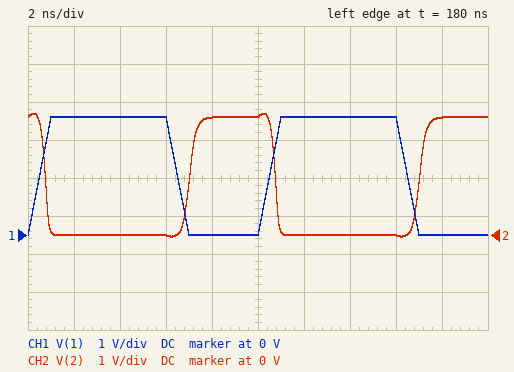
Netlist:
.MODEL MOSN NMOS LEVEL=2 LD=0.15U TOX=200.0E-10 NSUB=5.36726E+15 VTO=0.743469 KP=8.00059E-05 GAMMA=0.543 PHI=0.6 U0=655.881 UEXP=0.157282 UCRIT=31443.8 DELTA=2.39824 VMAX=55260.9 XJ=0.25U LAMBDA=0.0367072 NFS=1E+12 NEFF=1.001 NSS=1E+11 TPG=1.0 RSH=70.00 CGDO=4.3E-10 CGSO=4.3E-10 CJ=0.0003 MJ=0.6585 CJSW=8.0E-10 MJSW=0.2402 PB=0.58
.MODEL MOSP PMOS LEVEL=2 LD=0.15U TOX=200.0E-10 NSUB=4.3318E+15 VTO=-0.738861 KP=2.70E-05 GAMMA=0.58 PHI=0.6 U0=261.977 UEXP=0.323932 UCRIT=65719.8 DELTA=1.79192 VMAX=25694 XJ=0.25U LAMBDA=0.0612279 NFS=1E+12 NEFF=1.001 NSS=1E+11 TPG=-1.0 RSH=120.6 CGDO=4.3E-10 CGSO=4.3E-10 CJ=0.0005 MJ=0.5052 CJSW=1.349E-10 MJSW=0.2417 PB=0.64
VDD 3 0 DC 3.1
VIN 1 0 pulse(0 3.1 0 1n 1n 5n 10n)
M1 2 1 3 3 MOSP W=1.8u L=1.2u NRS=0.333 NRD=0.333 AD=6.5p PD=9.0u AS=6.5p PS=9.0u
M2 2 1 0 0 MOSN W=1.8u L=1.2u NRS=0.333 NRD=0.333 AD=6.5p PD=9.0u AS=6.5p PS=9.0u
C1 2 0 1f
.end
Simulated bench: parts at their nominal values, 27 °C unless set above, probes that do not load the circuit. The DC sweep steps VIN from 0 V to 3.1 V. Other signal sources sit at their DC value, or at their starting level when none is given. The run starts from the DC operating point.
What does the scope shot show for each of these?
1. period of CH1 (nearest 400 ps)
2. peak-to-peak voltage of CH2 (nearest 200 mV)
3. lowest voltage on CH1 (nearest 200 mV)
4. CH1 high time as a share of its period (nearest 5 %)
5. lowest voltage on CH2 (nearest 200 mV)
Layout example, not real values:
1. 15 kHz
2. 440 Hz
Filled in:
1. 10.0 ns
2. 3.2 V
3. 0 V
4. 60 %
5. 0 V
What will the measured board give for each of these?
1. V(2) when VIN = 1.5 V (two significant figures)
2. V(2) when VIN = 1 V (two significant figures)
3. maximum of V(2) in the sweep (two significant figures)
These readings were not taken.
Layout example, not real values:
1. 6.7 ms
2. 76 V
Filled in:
1. 210 mV
2. 2.9 V
3. 3.1 V
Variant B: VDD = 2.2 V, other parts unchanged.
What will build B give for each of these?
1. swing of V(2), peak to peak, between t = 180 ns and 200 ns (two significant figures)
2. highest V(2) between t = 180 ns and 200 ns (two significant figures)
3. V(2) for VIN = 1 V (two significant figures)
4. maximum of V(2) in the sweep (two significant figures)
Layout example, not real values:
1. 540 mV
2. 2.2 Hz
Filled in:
1. 2.4 V
2. 2.3 V
3. 750 mV
4. 2.2 V
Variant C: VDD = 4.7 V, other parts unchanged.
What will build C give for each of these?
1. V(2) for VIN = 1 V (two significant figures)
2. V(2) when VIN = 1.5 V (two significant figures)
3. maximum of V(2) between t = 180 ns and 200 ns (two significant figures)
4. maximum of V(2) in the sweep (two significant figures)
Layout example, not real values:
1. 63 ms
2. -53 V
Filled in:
1. 4.6 V
2. 4.1 V
3. 4.8 V
4. 4.7 V
